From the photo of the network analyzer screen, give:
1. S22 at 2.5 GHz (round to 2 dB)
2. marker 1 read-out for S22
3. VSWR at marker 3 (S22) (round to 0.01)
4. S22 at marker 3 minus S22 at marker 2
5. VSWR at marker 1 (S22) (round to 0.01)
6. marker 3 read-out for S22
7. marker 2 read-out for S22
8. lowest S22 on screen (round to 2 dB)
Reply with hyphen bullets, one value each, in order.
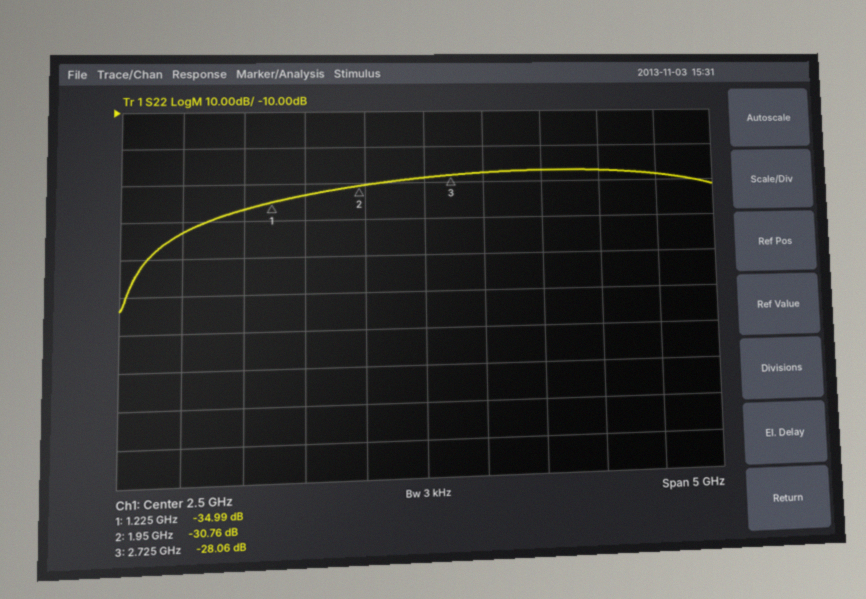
- -28 dB
- -34.99 dB
- 1.08
- 2.70 dB
- 1.04
- -28.06 dB
- -30.76 dB
- -64 dB
